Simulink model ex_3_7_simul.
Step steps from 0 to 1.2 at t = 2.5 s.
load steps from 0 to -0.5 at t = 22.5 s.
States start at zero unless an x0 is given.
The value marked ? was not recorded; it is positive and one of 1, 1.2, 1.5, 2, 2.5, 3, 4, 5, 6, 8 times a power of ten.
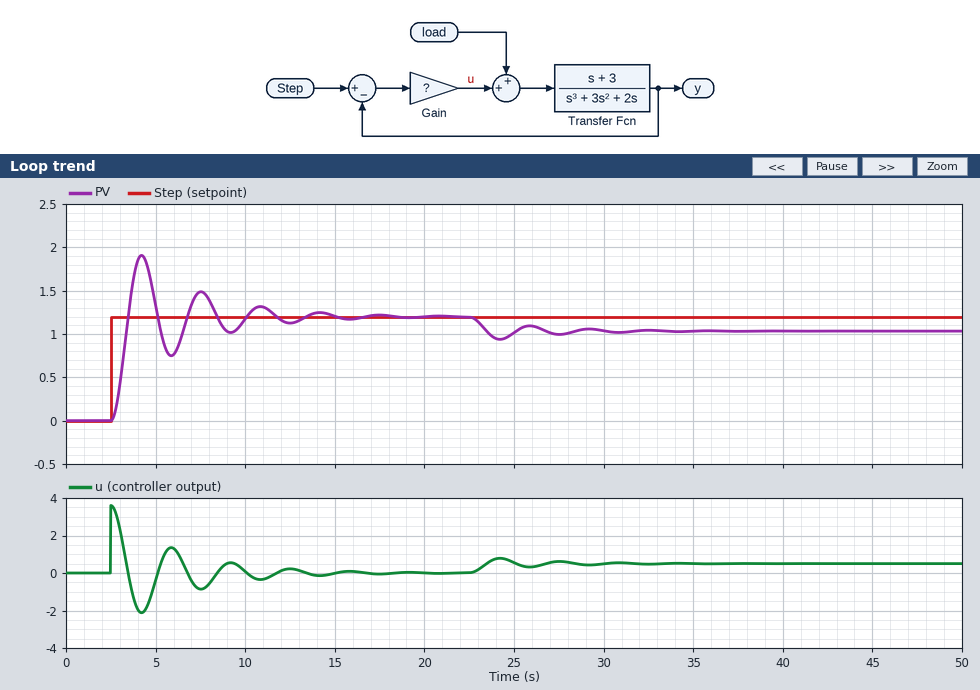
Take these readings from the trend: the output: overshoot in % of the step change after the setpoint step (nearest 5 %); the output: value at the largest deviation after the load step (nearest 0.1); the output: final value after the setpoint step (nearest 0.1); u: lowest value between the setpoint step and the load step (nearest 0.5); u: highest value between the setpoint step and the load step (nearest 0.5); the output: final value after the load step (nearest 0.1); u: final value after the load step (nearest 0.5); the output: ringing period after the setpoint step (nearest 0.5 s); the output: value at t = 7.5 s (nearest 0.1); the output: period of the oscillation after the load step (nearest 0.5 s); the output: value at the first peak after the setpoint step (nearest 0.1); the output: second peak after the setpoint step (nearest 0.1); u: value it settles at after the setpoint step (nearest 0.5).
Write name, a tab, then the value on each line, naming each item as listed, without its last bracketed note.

the output: overshoot in % of the step change after the setpoint step	60 %
the output: value at the largest deviation after the load step	0.9
the output: final value after the setpoint step	1.2
u: lowest value between the setpoint step and the load step	-2.0
u: highest value between the setpoint step and the load step	3.5
the output: final value after the load step	1.0
u: final value after the load step	0.5
the output: ringing period after the setpoint step	3.5 s
the output: value at t = 7.5 s	1.5
the output: period of the oscillation after the load step	3.5 s
the output: value at the first peak after the setpoint step	1.9
the output: second peak after the setpoint step	1.5
u: value it settles at after the setpoint step	0.0
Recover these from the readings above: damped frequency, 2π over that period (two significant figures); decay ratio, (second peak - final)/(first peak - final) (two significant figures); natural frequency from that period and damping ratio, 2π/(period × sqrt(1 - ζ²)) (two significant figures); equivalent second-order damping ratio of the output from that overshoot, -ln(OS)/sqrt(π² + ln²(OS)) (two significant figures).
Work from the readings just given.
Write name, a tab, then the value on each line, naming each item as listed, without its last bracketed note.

damped frequency, 2π over that period	1.8 rad/s
decay ratio, (second peak - final)/(first peak - final)	0.43
natural frequency from that period and damping ratio, 2π/(period × sqrt(1 - ζ²))	1.8 rad/s
equivalent second-order damping ratio of the output from that overshoot, -ln(OS)/sqrt(π² + ln²(OS))	0.16
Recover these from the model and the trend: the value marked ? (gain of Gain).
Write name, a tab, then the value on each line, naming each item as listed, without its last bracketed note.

the value marked ?	3
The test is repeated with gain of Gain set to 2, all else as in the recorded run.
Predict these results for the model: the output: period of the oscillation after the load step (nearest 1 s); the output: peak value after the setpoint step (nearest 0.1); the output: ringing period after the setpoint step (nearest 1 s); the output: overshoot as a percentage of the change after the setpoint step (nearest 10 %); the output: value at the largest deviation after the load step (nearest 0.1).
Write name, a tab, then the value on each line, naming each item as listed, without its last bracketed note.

the output: period of the oscillation after the load step	4 s
the output: peak value after the setpoint step	1.8
the output: ringing period after the setpoint step	4 s
the output: overshoot as a percentage of the change after the setpoint step	50 %
the output: value at the largest deviation after the load step	0.8
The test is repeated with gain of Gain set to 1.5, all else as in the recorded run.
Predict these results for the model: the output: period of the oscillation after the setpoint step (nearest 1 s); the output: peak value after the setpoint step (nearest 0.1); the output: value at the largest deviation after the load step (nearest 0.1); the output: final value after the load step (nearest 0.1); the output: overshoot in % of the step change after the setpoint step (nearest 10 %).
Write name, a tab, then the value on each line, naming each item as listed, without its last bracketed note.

the output: period of the oscillation after the setpoint step	5 s
the output: peak value after the setpoint step	1.7
the output: value at the largest deviation after the load step	0.7
the output: final value after the load step	0.9
the output: overshoot in % of the step change after the setpoint step	40 %
